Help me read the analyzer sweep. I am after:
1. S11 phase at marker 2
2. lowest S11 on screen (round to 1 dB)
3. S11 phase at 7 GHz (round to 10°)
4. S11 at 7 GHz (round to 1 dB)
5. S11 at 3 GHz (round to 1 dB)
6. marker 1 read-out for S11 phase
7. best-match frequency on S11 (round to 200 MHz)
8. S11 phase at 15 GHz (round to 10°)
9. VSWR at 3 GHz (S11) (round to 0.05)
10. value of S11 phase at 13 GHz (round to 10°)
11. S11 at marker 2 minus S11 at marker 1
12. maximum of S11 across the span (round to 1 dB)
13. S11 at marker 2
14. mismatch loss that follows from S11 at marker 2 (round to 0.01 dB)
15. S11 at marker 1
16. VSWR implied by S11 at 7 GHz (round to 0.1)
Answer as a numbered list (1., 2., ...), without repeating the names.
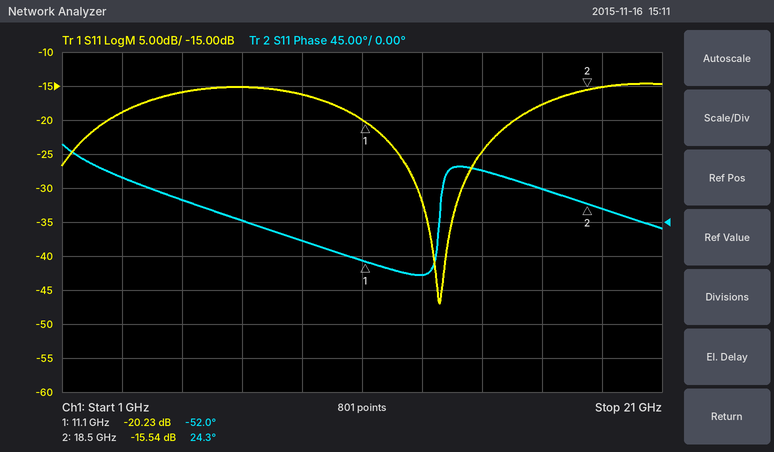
1. 24.3°
2. -47 dB
3. 0°
4. -15 dB
5. -19 dB
6. -52.0°
7. 13.6 GHz
8. 70°
9. 1.25
10. -70°
11. 4.69 dB
12. -15 dB
13. -15.54 dB
14. 0.12 dB
15. -20.23 dB
16. 1.4
